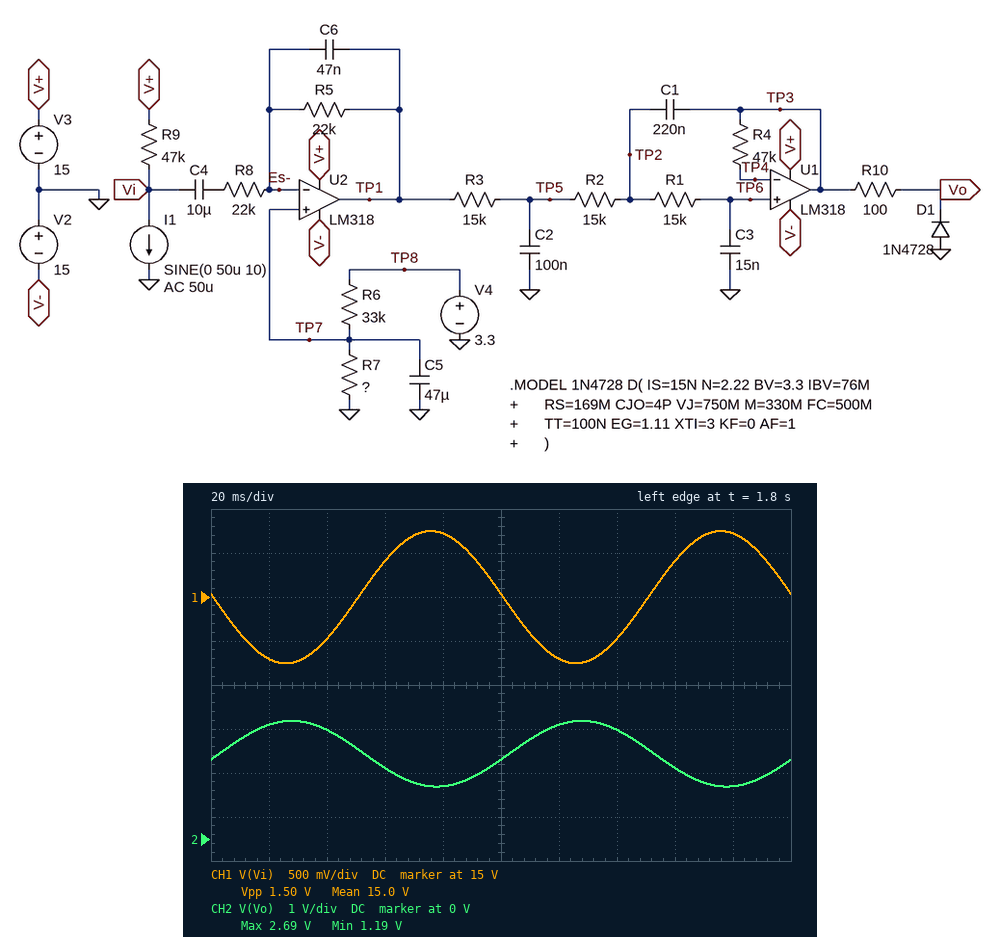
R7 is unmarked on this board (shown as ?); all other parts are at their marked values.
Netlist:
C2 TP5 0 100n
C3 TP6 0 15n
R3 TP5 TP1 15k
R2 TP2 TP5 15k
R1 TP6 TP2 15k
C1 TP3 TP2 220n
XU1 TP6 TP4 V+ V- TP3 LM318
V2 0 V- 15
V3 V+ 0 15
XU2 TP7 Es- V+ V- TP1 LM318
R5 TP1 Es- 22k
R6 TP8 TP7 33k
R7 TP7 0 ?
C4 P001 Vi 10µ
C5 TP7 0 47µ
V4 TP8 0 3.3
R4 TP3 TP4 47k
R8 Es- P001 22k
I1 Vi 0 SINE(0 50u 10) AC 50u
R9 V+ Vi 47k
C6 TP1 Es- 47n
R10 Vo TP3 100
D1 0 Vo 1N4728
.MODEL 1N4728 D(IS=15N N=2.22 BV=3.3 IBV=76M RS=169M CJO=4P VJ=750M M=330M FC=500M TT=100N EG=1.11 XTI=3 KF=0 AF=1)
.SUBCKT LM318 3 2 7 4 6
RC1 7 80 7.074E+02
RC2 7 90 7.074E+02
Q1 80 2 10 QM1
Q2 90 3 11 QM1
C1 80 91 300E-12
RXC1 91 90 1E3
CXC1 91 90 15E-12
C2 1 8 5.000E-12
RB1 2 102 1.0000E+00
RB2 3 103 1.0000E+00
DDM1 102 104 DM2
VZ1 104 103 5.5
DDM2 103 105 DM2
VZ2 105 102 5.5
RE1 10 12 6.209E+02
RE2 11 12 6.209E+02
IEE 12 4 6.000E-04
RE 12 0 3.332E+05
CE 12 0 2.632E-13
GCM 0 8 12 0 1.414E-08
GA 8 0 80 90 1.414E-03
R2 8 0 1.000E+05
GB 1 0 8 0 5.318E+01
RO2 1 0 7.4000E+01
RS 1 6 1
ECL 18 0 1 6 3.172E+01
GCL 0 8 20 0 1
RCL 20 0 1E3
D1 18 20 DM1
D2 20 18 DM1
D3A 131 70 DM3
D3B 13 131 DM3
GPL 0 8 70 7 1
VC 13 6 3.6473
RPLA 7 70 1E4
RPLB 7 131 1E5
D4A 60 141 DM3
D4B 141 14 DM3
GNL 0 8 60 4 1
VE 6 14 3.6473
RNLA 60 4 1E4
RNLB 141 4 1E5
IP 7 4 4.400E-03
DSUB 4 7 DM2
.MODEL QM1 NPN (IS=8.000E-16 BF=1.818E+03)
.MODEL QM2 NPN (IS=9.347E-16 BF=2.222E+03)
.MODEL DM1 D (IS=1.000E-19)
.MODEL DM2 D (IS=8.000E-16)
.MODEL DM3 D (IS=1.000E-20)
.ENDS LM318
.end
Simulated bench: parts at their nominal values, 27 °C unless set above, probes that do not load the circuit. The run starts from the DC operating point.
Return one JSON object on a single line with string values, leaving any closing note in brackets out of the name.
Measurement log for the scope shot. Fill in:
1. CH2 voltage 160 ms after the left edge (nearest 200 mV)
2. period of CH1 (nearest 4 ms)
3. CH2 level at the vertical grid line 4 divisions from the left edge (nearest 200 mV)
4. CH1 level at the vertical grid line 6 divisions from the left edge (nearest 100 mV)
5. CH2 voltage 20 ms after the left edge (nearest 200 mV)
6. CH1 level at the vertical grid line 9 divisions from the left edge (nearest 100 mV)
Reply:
{"CH2 voltage 160 ms after the left edge": "1.6 V", "period of CH1": "100 ms", "CH2 level at the vertical grid line 4 divisions from the left edge": "1.2 V", "CH1 level at the vertical grid line 6 divisions from the left edge": "14.3 V", "CH2 voltage 20 ms after the left edge": "2.6 V", "CH1 level at the vertical grid line 9 divisions from the left edge": "15.7 V"}
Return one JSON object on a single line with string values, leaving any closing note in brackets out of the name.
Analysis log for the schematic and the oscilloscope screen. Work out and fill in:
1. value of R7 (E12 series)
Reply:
{"value of R7": "47 kΩ"}
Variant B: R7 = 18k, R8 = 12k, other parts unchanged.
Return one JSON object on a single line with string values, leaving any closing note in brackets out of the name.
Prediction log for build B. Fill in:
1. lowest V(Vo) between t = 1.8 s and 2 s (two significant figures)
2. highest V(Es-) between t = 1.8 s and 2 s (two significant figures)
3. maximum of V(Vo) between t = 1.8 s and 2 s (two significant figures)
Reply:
{"lowest V(Vo) between t = 1.8 s and 2 s": "290 mV", "highest V(Es-) between t = 1.8 s and 2 s": "1.2 V", "maximum of V(Vo) between t = 1.8 s and 2 s": "2.0 V"}
